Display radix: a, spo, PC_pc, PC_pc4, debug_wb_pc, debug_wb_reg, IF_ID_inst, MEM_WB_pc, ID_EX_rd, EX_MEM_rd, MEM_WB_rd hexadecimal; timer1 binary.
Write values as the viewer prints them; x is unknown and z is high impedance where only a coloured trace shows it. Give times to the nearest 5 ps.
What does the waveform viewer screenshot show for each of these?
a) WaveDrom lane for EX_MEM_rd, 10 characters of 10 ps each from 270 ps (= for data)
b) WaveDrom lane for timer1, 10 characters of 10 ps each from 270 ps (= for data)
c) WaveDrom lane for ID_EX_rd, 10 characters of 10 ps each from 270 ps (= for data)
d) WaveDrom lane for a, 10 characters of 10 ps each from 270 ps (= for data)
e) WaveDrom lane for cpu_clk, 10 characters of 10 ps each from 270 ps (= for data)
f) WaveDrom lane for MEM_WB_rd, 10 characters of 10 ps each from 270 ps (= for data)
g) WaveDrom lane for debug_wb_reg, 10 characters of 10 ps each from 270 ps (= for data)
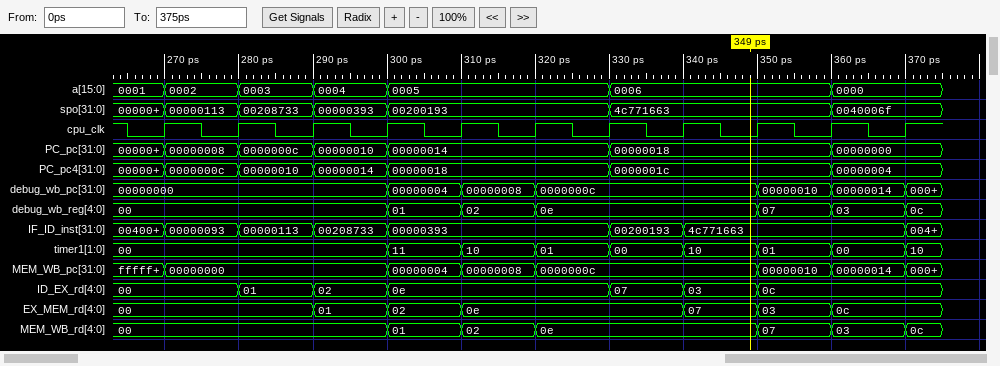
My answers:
{name: 'EX_MEM_rd', wave: '=.===..===', data: '00 01 02 0e 07 03 0c'}
{name: 'timer1', wave: '=..=======', data: '00 11 10 01 00 10 01 00'}
{name: 'ID_EX_rd', wave: '====..===.', data: '00 01 02 0e 07 03 0c'}
{name: 'a', wave: '====..=..=', data: '0002 0003 0004 0005 0006 0000'}
{name: 'cpu_clk', wave: 'p.........'}
{name: 'MEM_WB_rd', wave: '=..===..==', data: '00 01 02 0e 07 03'}
{name: 'debug_wb_reg', wave: '=..===..==', data: '00 01 02 0e 07 03'}
